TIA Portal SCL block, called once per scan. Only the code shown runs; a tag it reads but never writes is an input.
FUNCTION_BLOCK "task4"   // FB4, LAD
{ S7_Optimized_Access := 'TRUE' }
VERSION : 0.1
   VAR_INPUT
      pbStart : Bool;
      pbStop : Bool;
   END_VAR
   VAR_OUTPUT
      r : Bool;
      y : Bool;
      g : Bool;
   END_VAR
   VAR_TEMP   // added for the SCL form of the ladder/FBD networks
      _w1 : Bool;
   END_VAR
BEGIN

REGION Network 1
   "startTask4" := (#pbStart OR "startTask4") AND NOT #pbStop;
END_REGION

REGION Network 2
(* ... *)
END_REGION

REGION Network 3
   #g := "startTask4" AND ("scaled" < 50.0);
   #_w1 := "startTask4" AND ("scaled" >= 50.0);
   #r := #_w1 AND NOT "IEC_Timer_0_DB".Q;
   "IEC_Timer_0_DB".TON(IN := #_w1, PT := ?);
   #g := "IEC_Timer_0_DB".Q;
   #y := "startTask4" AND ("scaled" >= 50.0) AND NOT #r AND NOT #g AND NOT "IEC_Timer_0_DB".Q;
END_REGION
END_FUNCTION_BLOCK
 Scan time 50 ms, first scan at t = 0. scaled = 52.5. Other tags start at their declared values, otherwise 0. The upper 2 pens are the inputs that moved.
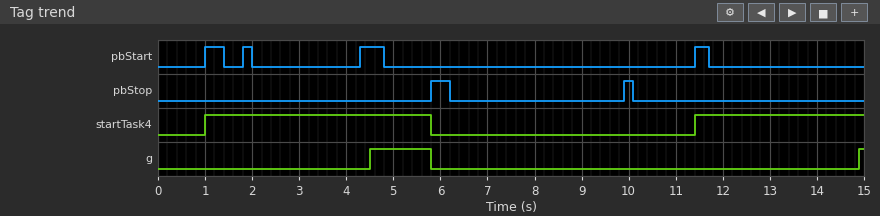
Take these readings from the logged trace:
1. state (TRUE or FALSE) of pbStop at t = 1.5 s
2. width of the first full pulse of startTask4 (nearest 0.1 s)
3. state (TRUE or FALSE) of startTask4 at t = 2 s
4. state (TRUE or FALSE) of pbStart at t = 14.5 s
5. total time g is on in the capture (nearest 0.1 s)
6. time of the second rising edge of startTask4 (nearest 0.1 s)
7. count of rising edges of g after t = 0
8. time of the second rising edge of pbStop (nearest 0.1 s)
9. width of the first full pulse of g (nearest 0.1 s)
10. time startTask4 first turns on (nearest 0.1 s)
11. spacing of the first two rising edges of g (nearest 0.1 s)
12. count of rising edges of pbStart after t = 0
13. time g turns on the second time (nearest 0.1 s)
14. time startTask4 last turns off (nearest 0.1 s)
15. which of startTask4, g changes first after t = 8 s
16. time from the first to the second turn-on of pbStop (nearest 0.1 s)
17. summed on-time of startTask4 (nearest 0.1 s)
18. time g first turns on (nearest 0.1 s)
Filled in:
FALSE
4.8 s
TRUE
FALSE
1.4 s
11.4 s
2
9.9 s
1.3 s
1.0 s
10.4 s
4
14.9 s
5.8 s
startTask4
4.1 s
8.4 s
4.5 s
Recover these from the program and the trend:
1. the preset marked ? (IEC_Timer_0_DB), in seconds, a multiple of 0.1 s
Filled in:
3.5 s
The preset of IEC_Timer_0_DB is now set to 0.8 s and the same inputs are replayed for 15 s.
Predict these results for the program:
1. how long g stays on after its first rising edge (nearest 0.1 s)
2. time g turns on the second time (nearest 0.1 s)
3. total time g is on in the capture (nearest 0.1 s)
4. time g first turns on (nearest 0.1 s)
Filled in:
4.0 s
12.2 s
6.8 s
1.8 s
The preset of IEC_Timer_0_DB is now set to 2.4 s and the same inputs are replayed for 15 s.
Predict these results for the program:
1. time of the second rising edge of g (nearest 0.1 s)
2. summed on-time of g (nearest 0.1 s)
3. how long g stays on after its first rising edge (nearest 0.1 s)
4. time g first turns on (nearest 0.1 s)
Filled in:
13.8 s
3.6 s
2.4 s
3.4 s
